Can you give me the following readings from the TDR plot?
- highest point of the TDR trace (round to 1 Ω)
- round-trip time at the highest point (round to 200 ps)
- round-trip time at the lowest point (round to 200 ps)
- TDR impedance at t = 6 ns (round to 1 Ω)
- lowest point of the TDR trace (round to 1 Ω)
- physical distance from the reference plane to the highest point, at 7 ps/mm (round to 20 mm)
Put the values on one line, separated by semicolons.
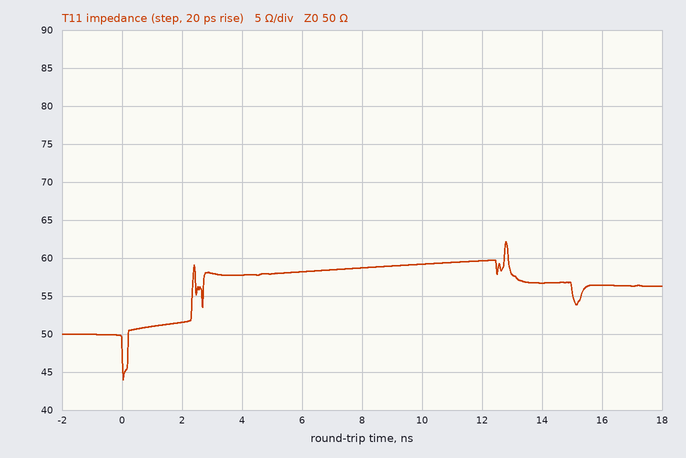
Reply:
62 Ω; 12.8 ns; 0.0 ns; 58 Ω; 44 Ω; 920 mm
